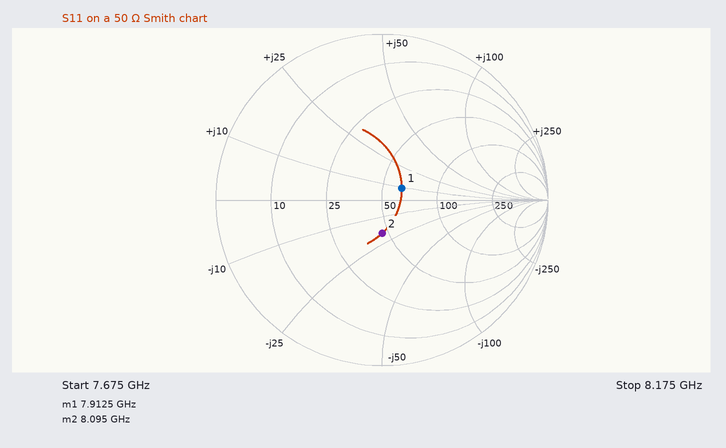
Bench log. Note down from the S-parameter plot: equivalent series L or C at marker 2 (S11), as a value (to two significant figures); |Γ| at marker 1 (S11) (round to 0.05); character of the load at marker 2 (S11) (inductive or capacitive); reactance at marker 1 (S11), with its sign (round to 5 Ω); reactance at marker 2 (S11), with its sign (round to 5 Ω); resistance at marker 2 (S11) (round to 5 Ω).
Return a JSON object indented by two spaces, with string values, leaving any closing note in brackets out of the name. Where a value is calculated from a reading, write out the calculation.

{
  "equivalent series L or C at marker 2 (S11), as a value": "C = 1/(2π × 8.095 GHz × 20 Ω) ≈ 1.0 pF",
  "|Γ| at marker 1 (S11)": "0.15",
  "character of the load at marker 2 (S11)": "capacitive",
  "reactance at marker 1 (S11), with its sign": "+10 Ω",
  "reactance at marker 2 (S11), with its sign": "-20 Ω",
  "resistance at marker 2 (S11)": "45 Ω"
}
